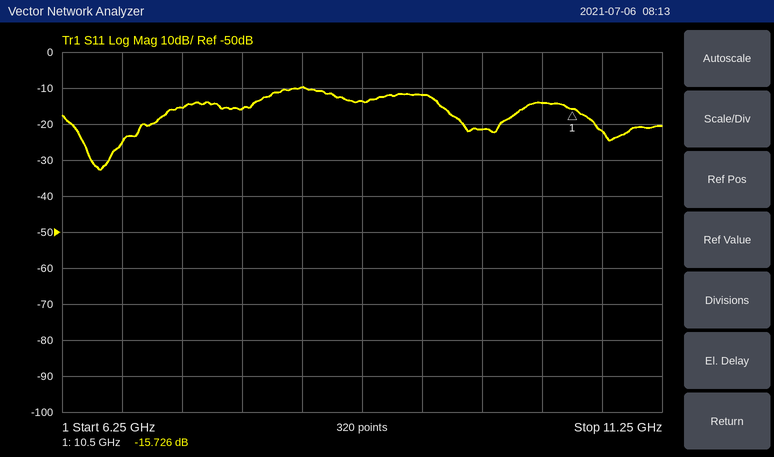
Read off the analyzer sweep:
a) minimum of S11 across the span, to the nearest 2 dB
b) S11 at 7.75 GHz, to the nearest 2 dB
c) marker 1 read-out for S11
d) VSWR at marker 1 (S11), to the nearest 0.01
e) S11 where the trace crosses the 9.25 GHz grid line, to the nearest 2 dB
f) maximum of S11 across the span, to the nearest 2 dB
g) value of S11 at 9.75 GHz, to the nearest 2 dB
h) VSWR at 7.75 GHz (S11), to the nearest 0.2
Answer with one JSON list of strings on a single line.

["-32 dB", "-16 dB", "-15.726 dB", "1.39", "-12 dB", "-10 dB", "-22 dB", "1.4"]
